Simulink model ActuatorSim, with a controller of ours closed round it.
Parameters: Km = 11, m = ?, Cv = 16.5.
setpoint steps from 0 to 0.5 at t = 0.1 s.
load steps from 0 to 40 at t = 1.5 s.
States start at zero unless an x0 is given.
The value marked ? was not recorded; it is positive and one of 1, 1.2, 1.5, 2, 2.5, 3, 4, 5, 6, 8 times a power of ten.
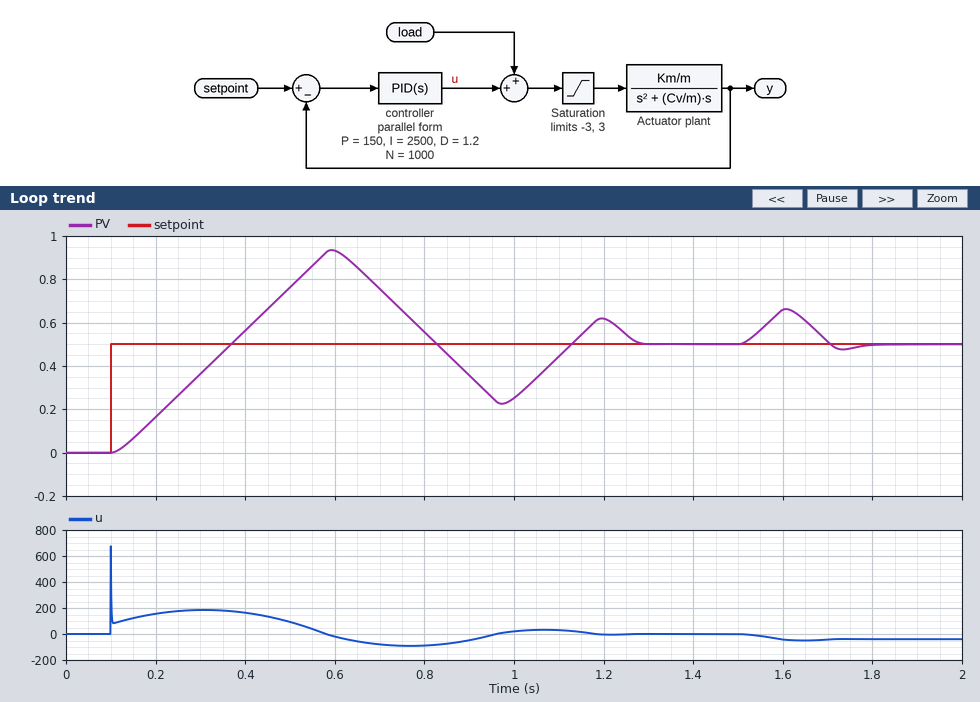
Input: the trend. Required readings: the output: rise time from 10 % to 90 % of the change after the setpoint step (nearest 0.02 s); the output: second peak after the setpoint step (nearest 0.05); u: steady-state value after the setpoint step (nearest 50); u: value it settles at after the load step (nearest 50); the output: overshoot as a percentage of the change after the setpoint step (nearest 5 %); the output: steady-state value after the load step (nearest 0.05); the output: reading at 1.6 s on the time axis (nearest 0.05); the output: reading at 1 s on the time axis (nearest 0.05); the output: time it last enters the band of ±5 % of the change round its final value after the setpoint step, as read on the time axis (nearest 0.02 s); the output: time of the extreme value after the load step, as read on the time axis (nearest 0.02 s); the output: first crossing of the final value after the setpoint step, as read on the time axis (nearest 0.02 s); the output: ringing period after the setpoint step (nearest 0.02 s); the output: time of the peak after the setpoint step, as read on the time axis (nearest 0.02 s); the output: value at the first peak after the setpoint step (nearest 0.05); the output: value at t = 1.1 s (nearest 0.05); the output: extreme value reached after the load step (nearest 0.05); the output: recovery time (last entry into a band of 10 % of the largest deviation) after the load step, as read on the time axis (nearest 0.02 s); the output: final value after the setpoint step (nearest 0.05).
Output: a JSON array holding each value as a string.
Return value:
["0.20 s", "0.60", "0", "-50", "85 %", "0.50", "0.65", "0.25", "1.26 s", "1.60 s", "0.36 s", "0.60 s", "0.60 s", "0.95", "0.45", "0.65", "1.76 s", "0.50"]
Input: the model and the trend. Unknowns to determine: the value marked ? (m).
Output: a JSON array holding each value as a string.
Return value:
["0.3"]
